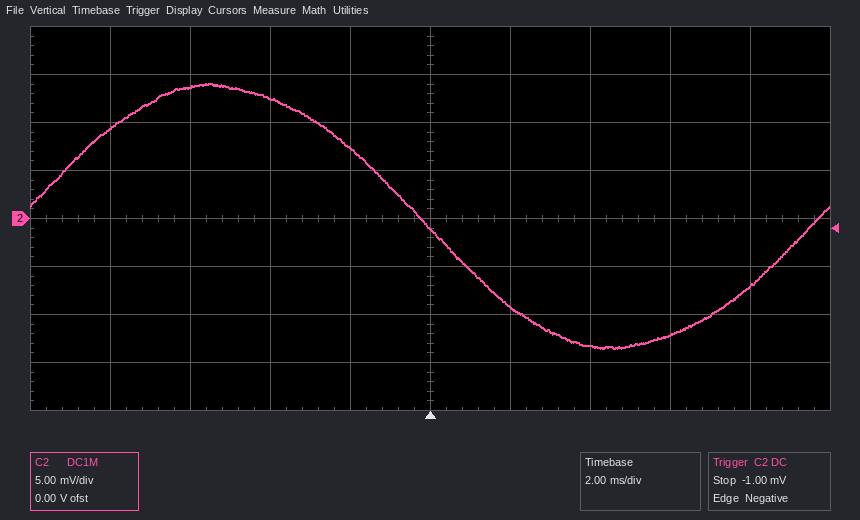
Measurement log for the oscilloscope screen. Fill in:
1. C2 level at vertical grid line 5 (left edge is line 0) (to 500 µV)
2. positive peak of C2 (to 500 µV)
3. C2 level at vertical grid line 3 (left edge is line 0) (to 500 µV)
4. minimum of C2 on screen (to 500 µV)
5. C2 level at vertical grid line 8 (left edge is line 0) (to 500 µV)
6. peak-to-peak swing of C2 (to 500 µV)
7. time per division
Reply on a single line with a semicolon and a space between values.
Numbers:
-1.0 mV; 14.0 mV; 12.5 mV; -13.5 mV; -12.0 mV; 27.5 mV; 2 ms
